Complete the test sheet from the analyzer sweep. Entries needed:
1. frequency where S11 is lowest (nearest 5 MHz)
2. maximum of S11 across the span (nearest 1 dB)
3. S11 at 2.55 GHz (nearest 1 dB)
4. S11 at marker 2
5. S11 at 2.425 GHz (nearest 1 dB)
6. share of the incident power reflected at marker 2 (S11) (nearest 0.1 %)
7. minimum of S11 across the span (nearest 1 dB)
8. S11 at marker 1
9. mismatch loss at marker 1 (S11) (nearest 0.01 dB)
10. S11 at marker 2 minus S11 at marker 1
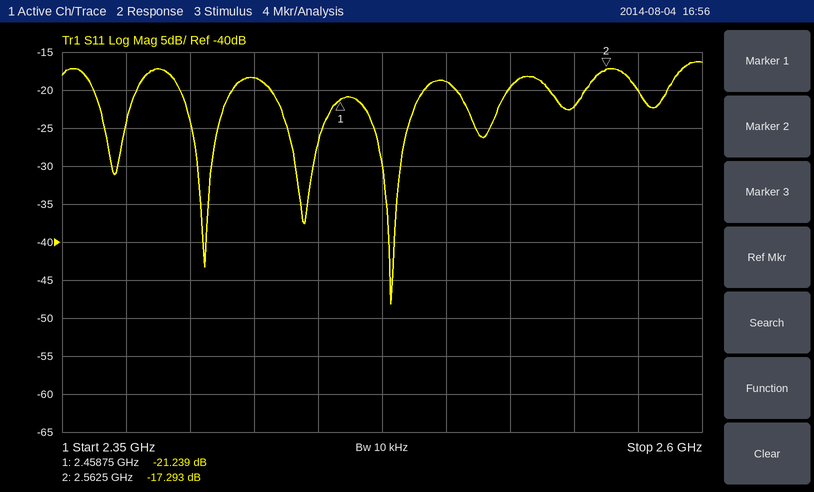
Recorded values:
2.480 GHz
-16 dB
-22 dB
-17.293 dB
-18 dB
1.9 %
-48 dB
-21.239 dB
0.03 dB
3.946 dB
